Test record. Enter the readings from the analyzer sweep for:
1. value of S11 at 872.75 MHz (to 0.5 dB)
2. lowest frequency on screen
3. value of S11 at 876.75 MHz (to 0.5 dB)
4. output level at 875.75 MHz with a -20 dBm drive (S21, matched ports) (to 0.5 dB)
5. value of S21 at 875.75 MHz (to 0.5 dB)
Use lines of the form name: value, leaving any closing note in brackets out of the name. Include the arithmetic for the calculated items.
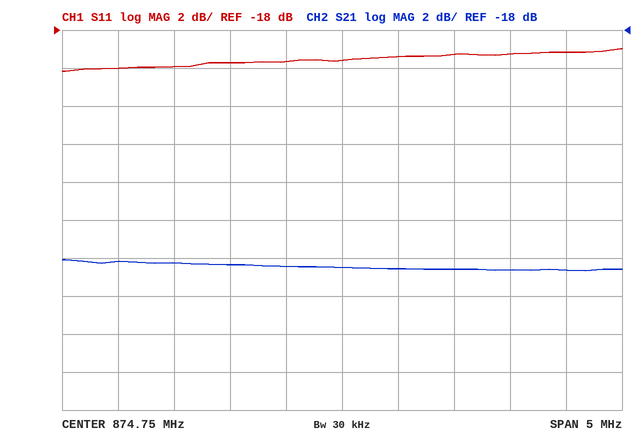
value of S11 at 872.75 MHz: -20.0 dB
lowest frequency on screen: 872.25 MHz
value of S11 at 876.75 MHz: -19.0 dB
output level at 875.75 MHz with a -20 dBm drive (S21, matched ports): -20 dBm + (-30.5 dB) = -50.5 dBm
value of S21 at 875.75 MHz: -30.5 dB
